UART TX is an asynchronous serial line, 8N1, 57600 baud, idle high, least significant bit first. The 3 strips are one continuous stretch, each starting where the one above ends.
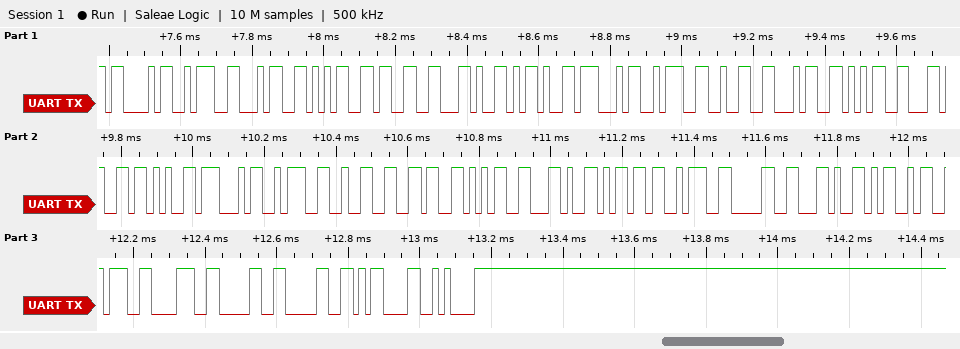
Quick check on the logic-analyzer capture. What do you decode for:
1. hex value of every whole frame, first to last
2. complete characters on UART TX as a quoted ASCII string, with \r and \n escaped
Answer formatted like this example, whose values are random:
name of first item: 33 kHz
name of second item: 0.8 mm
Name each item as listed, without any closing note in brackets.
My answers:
hex value of every whole frame, first to last: 43 3A 34 35 33 2C 2D 47 3A 32 34 35 2C 2B 47 3A 32 36 35 2C 6D 3A 30 2C 4D 3A 38 30 30 0D 0A
complete characters on UART TX as a quoted ASCII string, with \r and \n escaped: "C:453,-G:245,+G:265,m:0,M:800\r\n"
